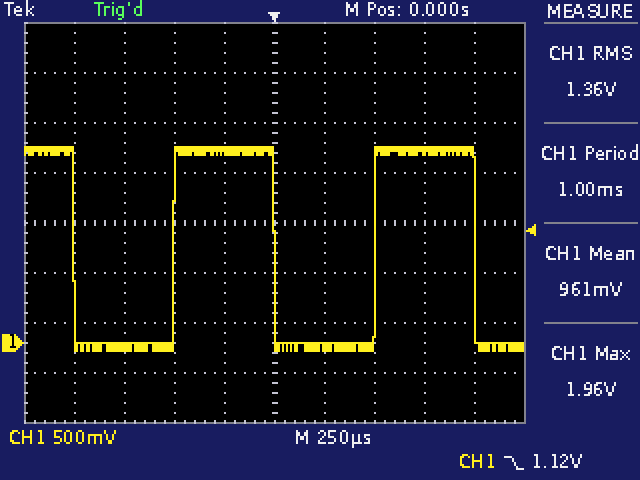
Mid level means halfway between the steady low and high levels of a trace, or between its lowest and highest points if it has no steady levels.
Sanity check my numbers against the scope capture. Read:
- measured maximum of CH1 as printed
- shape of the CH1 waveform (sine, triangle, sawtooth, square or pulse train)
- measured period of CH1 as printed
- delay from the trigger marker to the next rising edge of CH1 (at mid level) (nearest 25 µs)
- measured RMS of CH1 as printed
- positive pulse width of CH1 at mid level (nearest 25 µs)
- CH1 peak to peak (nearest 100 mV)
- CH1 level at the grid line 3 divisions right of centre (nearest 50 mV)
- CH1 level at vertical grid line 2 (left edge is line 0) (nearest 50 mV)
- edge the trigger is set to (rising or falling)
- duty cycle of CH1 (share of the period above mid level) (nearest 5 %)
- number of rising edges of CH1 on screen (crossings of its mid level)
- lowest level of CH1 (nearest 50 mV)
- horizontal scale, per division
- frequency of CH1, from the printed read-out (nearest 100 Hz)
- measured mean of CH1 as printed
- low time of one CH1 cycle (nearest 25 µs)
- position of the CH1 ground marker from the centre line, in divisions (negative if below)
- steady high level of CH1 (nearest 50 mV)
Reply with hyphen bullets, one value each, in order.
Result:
- 1.96 V
- square
- 1.00 ms
- 500 µs
- 1.36 V
- 500 µs
- 2.00 V
- 1.90 V
- -50 mV
- falling
- 50 %
- 2
- -100 mV
- 250 µs
- 1.0 kHz
- 961 mV
- 500 µs
- -2.4 div
- 1.90 V
